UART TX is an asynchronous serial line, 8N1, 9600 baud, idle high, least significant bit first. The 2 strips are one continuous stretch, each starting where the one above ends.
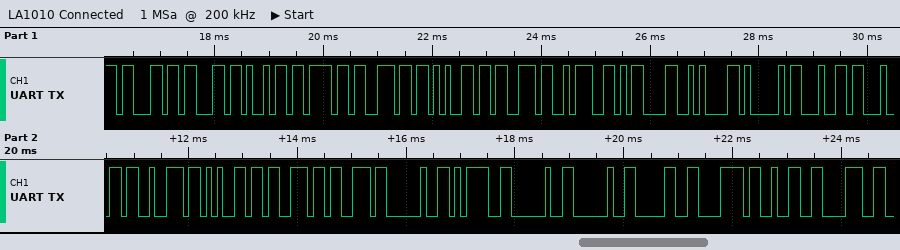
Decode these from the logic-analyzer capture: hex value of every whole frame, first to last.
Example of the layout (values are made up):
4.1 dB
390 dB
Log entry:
63 63 69 6F 6E 65 73 3A 0D 0A 41 64 64 72 65 73 73 20 3D 20 20 30 78 32 38
